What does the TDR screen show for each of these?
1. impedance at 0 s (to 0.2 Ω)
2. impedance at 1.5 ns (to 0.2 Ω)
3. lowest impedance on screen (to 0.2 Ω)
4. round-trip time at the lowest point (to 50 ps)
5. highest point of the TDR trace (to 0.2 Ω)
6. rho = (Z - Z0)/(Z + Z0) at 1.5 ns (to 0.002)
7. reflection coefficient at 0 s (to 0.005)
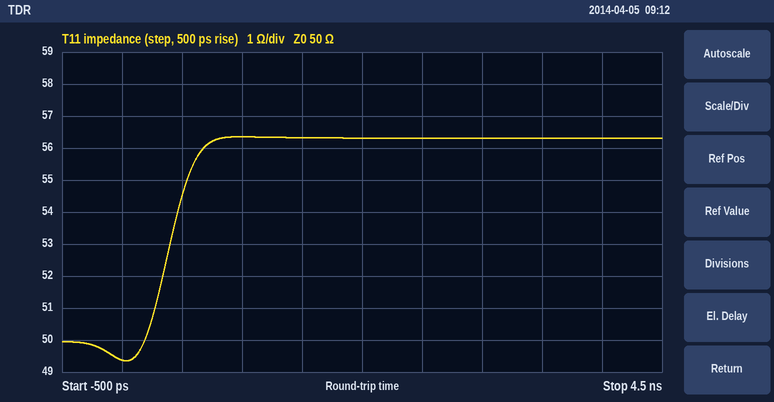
49.4 Ω
56.4 Ω
49.4 Ω
50 ps
56.4 Ω
+0.060
-0.005
